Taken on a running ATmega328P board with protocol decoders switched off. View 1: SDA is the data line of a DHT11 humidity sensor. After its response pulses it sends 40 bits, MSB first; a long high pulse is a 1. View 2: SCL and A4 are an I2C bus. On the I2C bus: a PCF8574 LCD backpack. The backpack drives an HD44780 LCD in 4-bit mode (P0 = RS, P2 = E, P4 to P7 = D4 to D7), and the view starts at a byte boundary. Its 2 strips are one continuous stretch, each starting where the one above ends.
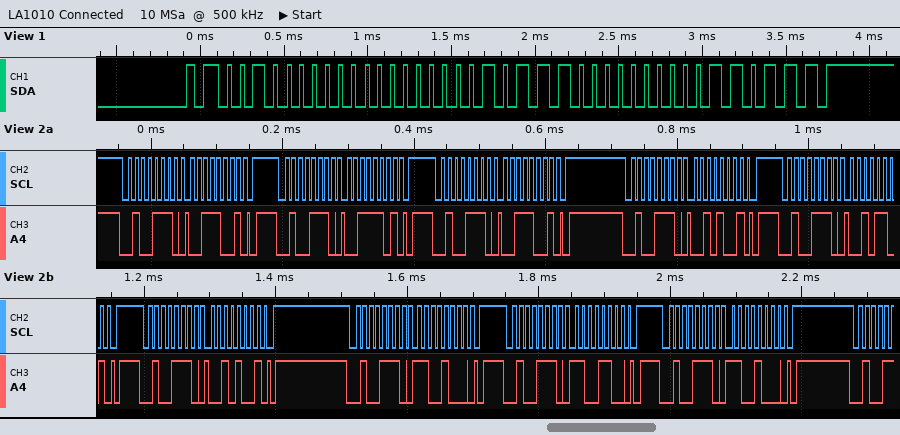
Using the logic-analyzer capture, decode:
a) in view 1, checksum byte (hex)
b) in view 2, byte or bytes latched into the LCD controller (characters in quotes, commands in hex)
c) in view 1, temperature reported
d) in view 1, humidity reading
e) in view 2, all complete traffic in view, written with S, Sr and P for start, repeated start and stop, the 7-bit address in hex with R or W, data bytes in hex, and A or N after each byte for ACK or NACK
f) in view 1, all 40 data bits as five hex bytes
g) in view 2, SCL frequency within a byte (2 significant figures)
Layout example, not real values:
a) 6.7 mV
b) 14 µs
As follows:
a) 0x37
b) '2'
c) 23.0 °C
d) 32 %
e) S 27W A 39 A P S 27W A 3D A P S 27W A 39 A P S 27W A 29 A P S 27W A 2D A P S 27W A 29 A P S 27W A C8 A P S 27W A CC A P S 27W A C8 A P
f) 20 00 17 00 37
g) 100 kHz
